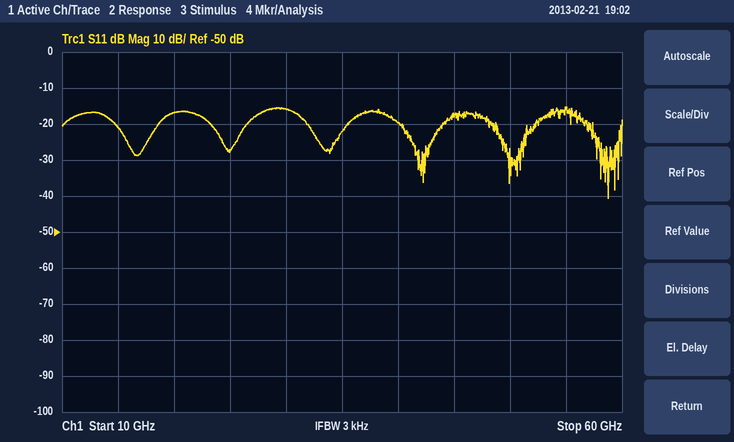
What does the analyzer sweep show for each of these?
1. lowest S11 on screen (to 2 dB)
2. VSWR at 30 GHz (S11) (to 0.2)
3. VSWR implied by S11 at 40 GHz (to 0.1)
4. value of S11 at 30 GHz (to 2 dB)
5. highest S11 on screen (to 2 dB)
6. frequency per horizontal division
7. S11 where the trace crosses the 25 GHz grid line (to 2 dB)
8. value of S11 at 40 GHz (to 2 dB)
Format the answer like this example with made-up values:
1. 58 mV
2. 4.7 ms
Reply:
1. -40 dB
2. 1.4
3. 1.2
4. -16 dB
5. -16 dB
6. 5 GHz
7. -28 dB
8. -20 dB
